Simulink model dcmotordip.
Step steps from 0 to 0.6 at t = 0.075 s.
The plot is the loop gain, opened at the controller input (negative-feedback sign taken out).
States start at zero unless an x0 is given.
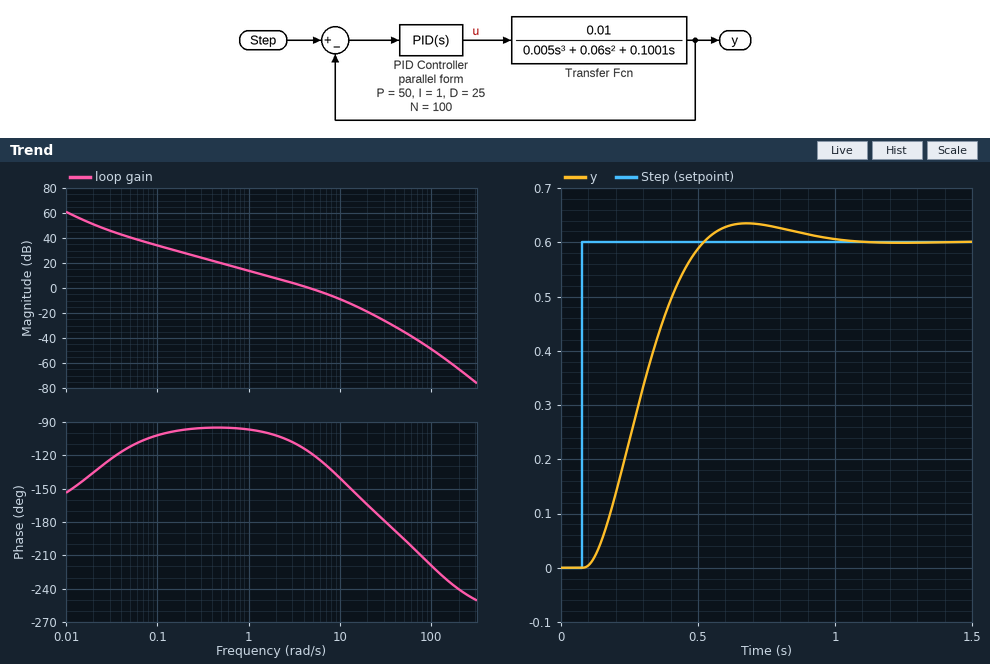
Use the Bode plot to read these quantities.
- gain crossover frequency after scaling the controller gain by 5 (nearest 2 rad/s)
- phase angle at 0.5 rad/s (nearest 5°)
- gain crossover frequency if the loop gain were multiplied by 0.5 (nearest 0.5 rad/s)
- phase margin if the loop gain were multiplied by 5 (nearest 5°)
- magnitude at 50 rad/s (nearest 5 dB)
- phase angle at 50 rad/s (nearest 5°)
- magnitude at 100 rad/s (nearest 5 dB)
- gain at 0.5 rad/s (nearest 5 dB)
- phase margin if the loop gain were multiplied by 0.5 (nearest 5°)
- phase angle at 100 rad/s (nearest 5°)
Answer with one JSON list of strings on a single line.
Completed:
["14 rad/s", "-95°", "2.5 rad/s", "25°", "-35 dB", "-195°", "-50 dB", "20 dB", "75°", "-220°"]
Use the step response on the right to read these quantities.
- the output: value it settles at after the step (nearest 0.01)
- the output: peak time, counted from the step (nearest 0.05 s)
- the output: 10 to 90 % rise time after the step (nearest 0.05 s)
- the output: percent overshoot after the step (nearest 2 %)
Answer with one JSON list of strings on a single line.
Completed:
["0.60", "0.60 s", "0.30 s", "6 %"]
